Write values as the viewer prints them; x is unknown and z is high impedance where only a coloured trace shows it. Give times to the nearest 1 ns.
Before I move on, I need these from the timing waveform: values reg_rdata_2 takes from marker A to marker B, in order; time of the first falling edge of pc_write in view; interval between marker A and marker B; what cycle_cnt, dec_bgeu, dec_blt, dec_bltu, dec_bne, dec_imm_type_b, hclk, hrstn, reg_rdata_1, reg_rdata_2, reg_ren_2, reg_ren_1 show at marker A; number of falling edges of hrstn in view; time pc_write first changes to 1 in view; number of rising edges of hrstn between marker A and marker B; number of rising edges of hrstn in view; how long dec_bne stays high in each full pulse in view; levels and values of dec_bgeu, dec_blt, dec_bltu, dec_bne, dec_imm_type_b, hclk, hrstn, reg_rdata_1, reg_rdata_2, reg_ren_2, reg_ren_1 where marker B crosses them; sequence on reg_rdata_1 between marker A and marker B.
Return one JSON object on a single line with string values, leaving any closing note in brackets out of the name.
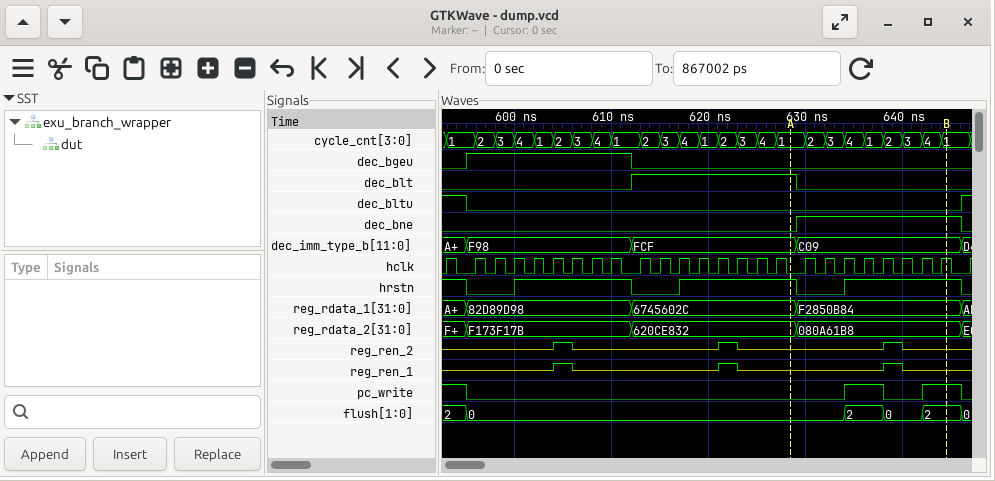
{"values reg_rdata_2 takes from marker A to marker B, in order": "620CE832, 080A61B8", "time of the first falling edge of pc_write in view": "595 ns", "interval between marker A and marker B": "16 ns", "what cycle_cnt, dec_bgeu, dec_blt, dec_bltu, dec_bne, dec_imm_type_b, hclk, hrstn, reg_rdata_1, reg_rdata_2, reg_ren_2, reg_ren_1 show at marker A": "cycle_cnt=1, dec_bgeu=0, dec_blt=1, dec_bltu=0, dec_bne=0, dec_imm_type_b=FCF, hclk=0, hrstn=1, reg_rdata_1=6745602C, reg_rdata_2=620CE832, reg_ren_2=z, reg_ren_1=z", "number of falling edges of hrstn in view": "4", "time pc_write first changes to 1 in view": "634 ns", "number of rising edges of hrstn between marker A and marker B": "1", "number of rising edges of hrstn in view": "3", "how long dec_bne stays high in each full pulse in view": "17 ns", "levels and values of dec_bgeu, dec_blt, dec_bltu, dec_bne, dec_imm_type_b, hclk, hrstn, reg_rdata_1, reg_rdata_2, reg_ren_2, reg_ren_1 where marker B crosses them": "dec_bgeu=0, dec_blt=0, dec_bltu=0, dec_bne=1, dec_imm_type_b=C09, hclk=1, hrstn=1, reg_rdata_1=F2850B84, reg_rdata_2=080A61B8, reg_ren_2=z, reg_ren_1=z", "sequence on reg_rdata_1 between marker A and marker B": "6745602C, F2850B84"}
